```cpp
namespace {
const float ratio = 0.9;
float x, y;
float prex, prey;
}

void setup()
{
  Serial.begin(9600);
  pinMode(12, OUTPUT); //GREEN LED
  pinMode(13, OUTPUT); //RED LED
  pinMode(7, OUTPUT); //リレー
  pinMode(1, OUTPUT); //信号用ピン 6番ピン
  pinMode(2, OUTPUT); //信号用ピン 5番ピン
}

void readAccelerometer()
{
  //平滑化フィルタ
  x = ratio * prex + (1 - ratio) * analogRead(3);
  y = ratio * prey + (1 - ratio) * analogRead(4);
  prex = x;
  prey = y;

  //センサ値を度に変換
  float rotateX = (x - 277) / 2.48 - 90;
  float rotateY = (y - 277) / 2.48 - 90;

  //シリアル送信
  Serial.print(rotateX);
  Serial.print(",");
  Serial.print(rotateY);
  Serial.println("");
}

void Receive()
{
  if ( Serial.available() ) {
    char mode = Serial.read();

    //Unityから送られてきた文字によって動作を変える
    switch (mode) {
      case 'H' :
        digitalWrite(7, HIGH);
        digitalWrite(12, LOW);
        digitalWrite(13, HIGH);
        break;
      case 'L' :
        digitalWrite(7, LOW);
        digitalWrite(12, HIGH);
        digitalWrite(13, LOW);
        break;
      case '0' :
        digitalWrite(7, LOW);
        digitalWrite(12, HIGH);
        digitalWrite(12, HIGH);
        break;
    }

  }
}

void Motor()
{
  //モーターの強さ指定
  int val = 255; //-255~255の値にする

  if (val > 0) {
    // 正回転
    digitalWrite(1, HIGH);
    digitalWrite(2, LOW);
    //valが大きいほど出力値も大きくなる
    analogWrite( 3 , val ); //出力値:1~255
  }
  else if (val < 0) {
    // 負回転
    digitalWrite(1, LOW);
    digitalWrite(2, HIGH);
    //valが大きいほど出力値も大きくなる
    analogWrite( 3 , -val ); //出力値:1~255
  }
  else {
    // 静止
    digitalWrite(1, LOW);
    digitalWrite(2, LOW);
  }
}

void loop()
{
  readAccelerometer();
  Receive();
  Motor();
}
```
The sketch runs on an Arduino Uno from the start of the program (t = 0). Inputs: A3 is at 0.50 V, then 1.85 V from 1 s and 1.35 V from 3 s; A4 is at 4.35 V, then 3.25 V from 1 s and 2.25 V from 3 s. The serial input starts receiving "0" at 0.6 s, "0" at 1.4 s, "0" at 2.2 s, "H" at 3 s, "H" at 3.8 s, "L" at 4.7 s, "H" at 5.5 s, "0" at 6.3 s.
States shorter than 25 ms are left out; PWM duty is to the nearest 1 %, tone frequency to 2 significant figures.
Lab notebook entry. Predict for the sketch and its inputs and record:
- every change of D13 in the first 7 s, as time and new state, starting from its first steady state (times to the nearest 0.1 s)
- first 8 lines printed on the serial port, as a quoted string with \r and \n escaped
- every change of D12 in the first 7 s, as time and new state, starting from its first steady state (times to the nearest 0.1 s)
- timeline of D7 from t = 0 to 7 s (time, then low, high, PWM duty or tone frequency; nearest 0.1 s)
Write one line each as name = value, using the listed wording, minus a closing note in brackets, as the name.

every change of D13 in the first 7 s, as time and new state, starting from its first steady state = 0 s low; 3 s high; 4.7 s low; 5.5 s high
first 8 lines printed on the serial port, as a quoted string with \r and \n escaped = "-197.58,-165.81\r\n-193.88,-133.51\r\n-190.55,-104.44\r\n-187.55,-78.28\r\n-184.85,-54.73\r\n-182.42,-33.54\r\n-180.24,-14.47\r\n-178.27,2.70\r\n"
every change of D12 in the first 7 s, as time and new state, starting from its first steady state = 0 s low; 0.6 s high; 3 s low; 4.7 s high; 5.5 s low; 6.3 s high
timeline of D7 from t = 0 to 7 s = 0 s low; 3 s high; 4.7 s low; 5.5 s high; 6.3 s low
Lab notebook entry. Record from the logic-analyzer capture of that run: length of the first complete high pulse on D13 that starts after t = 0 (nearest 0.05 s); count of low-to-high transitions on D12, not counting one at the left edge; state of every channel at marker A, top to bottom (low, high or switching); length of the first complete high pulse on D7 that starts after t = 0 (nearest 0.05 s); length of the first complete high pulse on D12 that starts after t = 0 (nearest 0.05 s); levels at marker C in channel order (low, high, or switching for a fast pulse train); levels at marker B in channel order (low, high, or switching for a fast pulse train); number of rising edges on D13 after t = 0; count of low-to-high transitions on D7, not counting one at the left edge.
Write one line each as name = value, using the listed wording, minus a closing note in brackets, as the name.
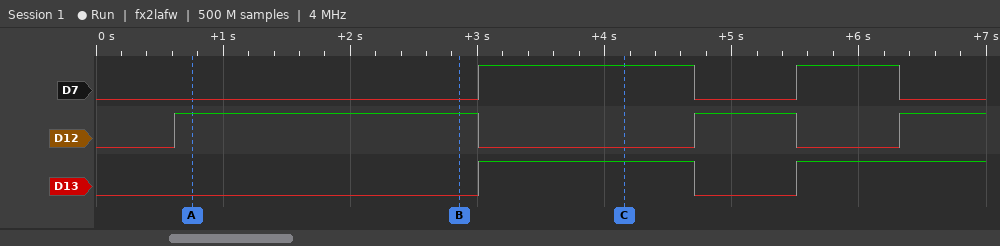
length of the first complete high pulse on D13 that starts after t = 0 = 1.70 s
count of low-to-high transitions on D12, not counting one at the left edge = 3
state of every channel at marker A, top to bottom = D7 low, D12 high, D13 low
length of the first complete high pulse on D7 that starts after t = 0 = 1.70 s
length of the first complete high pulse on D12 that starts after t = 0 = 2.40 s
levels at marker C in channel order = D7 high, D12 low, D13 high
levels at marker B in channel order = D7 low, D12 high, D13 low
number of rising edges on D13 after t = 0 = 2
count of low-to-high transitions on D7, not counting one at the left edge = 2
